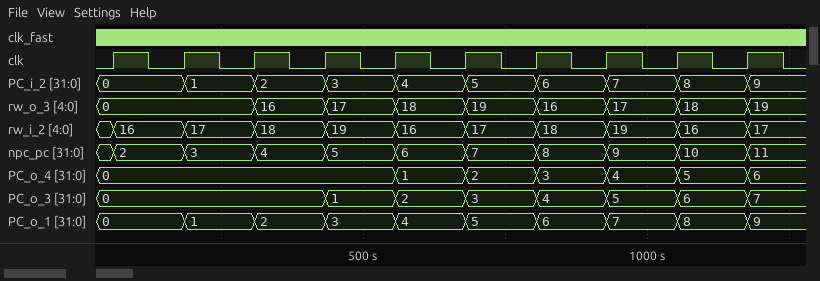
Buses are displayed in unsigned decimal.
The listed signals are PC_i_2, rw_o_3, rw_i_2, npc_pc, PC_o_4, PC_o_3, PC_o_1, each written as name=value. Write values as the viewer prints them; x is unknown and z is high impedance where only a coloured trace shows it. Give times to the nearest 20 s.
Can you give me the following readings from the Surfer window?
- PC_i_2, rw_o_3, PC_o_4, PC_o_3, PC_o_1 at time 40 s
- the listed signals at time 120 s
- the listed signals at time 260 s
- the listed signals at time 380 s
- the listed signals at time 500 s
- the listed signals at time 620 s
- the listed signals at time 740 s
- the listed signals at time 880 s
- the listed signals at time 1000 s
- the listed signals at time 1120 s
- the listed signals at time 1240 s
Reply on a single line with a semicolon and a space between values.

PC_i_2=0, rw_o_3=0, PC_o_4=0, PC_o_3=0, PC_o_1=0; PC_i_2=0, rw_o_3=0, rw_i_2=16, npc_pc=2, PC_o_4=0, PC_o_3=0, PC_o_1=0; PC_i_2=1, rw_o_3=0, rw_i_2=17, npc_pc=3, PC_o_4=0, PC_o_3=0, PC_o_1=1; PC_i_2=2, rw_o_3=16, rw_i_2=18, npc_pc=4, PC_o_4=0, PC_o_3=0, PC_o_1=2; PC_i_2=3, rw_o_3=17, rw_i_2=19, npc_pc=5, PC_o_4=0, PC_o_3=1, PC_o_1=3; PC_i_2=4, rw_o_3=18, rw_i_2=16, npc_pc=6, PC_o_4=1, PC_o_3=2, PC_o_1=4; PC_i_2=5, rw_o_3=19, rw_i_2=17, npc_pc=7, PC_o_4=2, PC_o_3=3, PC_o_1=5; PC_i_2=6, rw_o_3=16, rw_i_2=18, npc_pc=8, PC_o_4=3, PC_o_3=4, PC_o_1=6; PC_i_2=7, rw_o_3=17, rw_i_2=19, npc_pc=9, PC_o_4=4, PC_o_3=5, PC_o_1=7; PC_i_2=8, rw_o_3=18, rw_i_2=16, npc_pc=10, PC_o_4=5, PC_o_3=6, PC_o_1=8; PC_i_2=9, rw_o_3=19, rw_i_2=17, npc_pc=11, PC_o_4=6, PC_o_3=7, PC_o_1=9
